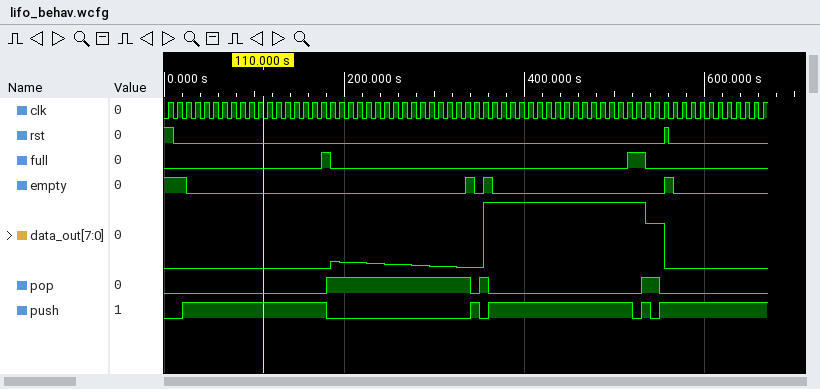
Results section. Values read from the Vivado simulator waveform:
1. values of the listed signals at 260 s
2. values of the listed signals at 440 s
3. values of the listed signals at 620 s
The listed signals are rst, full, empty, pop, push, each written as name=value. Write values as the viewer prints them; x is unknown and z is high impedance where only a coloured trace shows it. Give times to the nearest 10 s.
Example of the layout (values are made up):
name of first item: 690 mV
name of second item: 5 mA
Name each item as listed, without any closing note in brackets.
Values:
values of the listed signals at 260 s: rst=0, full=0, empty=0, pop=1, push=0
values of the listed signals at 440 s: rst=0, full=0, empty=0, pop=0, push=1
values of the listed signals at 620 s: rst=0, full=0, empty=0, pop=0, push=1
